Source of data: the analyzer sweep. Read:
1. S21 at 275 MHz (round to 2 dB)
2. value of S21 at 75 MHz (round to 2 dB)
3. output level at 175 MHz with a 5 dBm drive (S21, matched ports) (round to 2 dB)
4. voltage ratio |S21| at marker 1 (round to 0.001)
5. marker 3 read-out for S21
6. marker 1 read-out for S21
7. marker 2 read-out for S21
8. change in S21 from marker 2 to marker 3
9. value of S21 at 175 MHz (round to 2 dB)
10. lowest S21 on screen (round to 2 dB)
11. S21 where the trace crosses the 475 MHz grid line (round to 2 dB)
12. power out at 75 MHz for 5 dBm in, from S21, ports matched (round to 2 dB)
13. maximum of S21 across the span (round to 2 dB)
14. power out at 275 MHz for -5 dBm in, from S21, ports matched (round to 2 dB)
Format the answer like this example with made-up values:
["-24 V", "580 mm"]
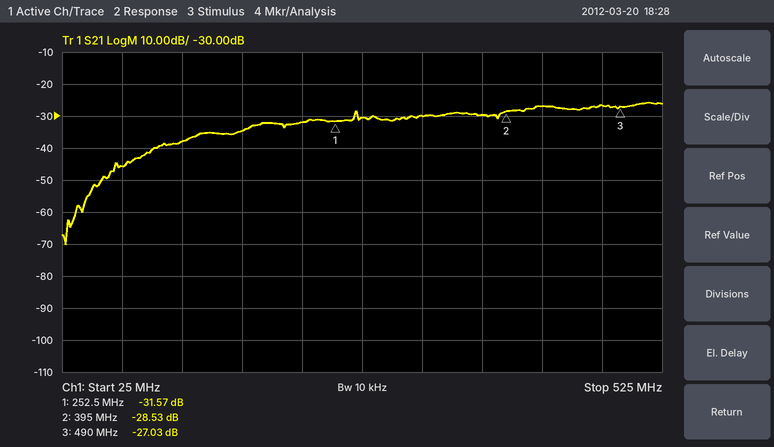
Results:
["-30 dB", "-46 dB", "-30 dBm", "0.026", "-27.03 dB", "-31.57 dB", "-28.53 dB", "1.50 dB", "-34 dB", "-70 dB", "-26 dB", "-40 dBm", "-26 dB", "-36 dBm"]
